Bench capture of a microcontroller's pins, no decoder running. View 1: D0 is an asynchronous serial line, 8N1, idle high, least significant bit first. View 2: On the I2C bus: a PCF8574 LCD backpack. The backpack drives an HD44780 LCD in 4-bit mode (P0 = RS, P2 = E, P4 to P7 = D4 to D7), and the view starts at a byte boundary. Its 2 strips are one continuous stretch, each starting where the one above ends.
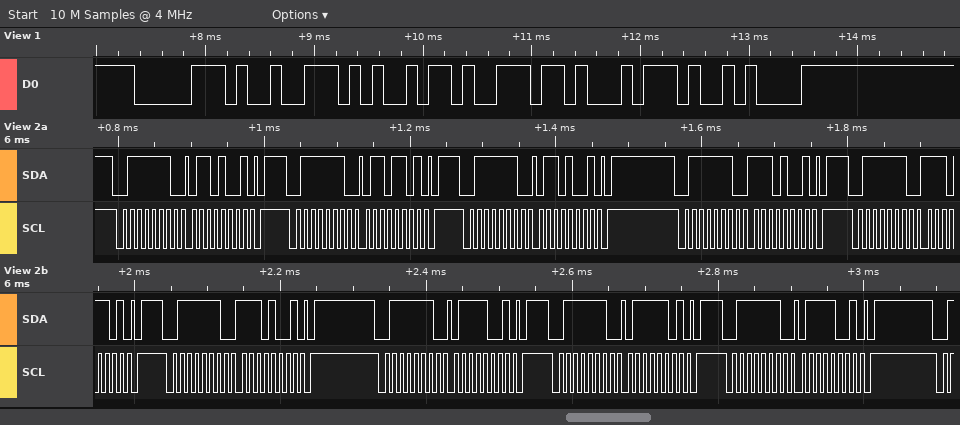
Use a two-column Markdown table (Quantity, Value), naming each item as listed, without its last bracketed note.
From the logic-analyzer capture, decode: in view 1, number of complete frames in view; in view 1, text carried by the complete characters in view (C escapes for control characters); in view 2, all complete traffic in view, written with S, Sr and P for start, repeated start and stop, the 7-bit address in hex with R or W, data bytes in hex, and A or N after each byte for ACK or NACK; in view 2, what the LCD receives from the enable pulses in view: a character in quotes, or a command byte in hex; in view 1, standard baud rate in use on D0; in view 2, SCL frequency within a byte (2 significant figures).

| Quantity | Value |
|---|---|
| in view 1, number of complete frames in view | 6 |
| in view 1, text carried by the complete characters in view | "print\n" |
| in view 2, all complete traffic in view, written with S, Sr and P for start, repeated start and stop, the 7-bit address in hex with R or W, data bytes in hex, and A or N after each byte for ACK or NACK | S 3FW A 69 A P S 3FW A 6D A P S 3FW A 69 A P S 3FW A E9 A P S 3FW A ED A P S 3FW A E9 A P S 3FW A 79 A P S 3FW A 7D A P S 3FW A 79 A P |
| in view 2, what the LCD receives from the enable pulses in view: a character in quotes, or a command byte in hex | 'n' |
| in view 1, standard baud rate in use on D0 | 9600 baud |
| in view 2, SCL frequency within a byte | 100 kHz |
